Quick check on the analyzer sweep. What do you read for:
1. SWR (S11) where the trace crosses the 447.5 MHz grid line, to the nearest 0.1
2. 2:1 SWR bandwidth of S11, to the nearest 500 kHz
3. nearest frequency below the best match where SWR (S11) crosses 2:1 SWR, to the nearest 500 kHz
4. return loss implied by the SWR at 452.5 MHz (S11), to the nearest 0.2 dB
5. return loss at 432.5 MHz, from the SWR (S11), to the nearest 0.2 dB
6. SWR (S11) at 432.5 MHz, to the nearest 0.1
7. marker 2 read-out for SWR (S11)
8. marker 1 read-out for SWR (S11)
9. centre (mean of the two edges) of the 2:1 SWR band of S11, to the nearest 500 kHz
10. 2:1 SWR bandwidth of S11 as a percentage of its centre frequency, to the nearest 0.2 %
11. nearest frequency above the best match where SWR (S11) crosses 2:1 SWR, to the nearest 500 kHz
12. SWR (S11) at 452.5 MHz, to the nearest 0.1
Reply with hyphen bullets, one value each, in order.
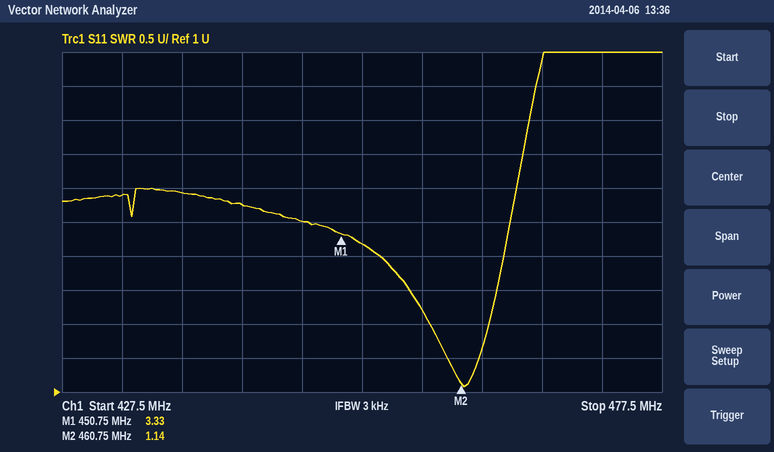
- 3.5
- 5.0 MHz
- 458.0 MHz
- 5.6 dB
- 4.6 dB
- 3.9
- 1.14
- 3.33
- 460.5 MHz
- 1.0 %
- 463.0 MHz
- 3.2
